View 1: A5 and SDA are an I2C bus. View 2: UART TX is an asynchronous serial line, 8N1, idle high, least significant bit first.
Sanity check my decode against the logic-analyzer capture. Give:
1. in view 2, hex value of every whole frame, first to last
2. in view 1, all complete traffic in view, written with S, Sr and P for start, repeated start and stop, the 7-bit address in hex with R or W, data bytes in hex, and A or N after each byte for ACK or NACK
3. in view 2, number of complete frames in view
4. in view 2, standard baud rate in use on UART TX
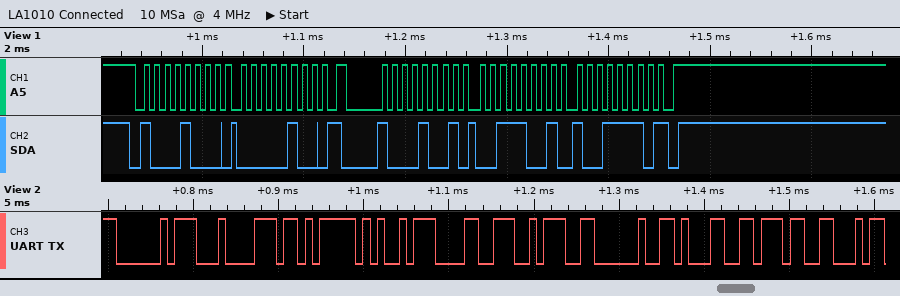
0xA0 0x84 0xEB 0xA5 0x98 0x3A 0x20 0x31 0x37
S 44W A 04 A Sr 44R A 39 A 9E N P
9
115200 baud
